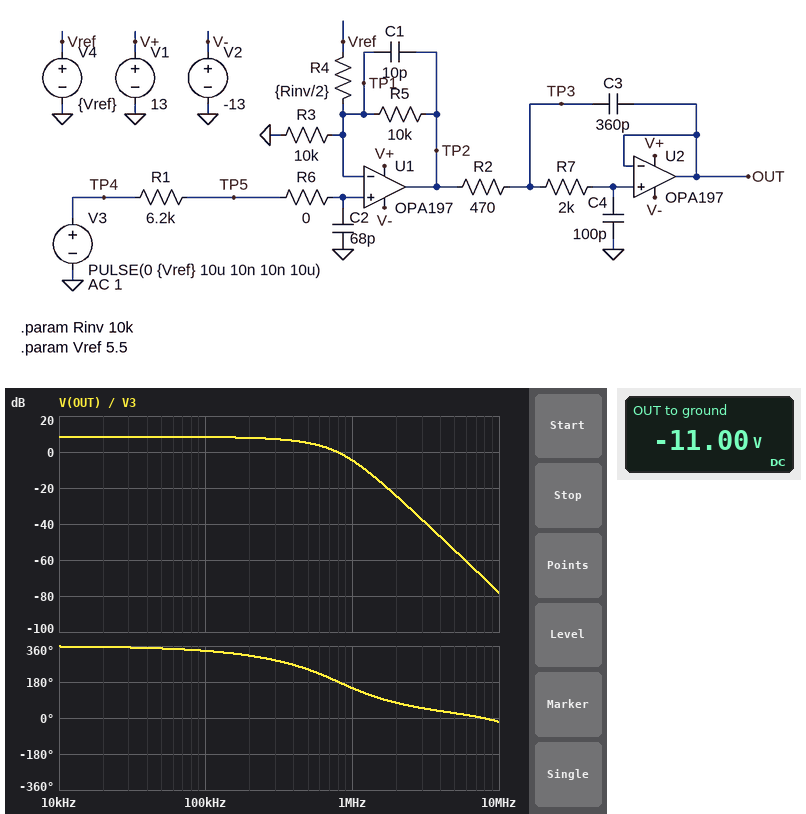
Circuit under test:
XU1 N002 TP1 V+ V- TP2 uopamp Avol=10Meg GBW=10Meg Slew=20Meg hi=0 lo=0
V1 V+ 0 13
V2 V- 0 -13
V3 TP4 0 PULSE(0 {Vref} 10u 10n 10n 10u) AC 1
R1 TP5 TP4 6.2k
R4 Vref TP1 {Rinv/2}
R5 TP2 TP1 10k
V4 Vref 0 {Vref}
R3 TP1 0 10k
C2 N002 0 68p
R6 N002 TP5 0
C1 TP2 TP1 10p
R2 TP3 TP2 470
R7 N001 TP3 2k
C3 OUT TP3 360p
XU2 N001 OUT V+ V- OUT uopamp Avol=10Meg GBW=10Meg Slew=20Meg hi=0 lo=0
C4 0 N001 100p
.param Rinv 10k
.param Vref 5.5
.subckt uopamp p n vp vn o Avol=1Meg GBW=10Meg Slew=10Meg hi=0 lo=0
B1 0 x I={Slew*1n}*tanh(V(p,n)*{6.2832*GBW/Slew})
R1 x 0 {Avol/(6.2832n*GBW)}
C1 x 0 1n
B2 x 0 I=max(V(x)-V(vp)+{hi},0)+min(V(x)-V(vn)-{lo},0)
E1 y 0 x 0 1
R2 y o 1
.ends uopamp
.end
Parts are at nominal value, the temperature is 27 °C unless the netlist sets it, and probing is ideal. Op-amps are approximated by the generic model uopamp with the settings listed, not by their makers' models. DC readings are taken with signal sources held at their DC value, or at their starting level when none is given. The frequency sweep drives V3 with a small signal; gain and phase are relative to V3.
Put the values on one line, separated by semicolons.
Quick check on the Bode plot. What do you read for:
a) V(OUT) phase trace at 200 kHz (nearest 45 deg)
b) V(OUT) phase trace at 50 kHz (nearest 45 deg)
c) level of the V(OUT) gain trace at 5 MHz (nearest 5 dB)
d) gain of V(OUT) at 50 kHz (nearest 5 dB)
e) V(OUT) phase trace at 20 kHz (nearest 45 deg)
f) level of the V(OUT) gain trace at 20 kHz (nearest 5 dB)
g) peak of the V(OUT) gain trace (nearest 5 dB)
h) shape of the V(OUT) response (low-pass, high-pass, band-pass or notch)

315 deg; 360 deg; -55 dB; 10 dB; 360 deg; 10 dB; 10 dB; low-pass
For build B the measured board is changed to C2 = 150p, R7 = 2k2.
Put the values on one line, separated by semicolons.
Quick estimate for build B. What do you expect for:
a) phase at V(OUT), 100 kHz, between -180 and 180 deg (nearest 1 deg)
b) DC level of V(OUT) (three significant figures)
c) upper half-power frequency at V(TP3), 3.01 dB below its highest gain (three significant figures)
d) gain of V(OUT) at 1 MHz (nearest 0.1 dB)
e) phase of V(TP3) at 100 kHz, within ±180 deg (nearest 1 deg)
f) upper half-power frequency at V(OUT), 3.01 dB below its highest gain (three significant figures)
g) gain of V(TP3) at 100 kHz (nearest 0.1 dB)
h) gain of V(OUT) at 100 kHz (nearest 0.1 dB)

-36 deg; -11.0 V; 280 kHz; -11.4 dB; -28 deg; 248 kHz; 7.9 dB; 7.8 dB
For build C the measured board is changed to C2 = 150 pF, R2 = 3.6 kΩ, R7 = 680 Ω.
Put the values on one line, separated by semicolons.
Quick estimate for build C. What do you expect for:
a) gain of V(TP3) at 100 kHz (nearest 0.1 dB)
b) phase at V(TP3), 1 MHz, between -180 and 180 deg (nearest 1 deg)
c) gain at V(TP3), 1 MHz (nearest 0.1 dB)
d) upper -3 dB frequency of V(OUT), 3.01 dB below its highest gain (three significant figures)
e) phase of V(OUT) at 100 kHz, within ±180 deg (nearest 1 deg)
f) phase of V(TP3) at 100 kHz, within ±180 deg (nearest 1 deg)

7.9 dB; 129 deg; -18.3 dB; 248 kHz; -42 deg; -39 deg
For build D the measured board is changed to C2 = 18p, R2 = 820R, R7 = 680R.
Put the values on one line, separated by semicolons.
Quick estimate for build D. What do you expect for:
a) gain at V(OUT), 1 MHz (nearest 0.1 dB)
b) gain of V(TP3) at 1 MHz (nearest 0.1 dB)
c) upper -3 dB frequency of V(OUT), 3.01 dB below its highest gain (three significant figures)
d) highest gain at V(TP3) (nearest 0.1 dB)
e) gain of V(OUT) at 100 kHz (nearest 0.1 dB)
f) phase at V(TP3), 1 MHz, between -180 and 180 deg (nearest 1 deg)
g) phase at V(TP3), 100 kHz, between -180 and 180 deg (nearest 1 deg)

5.1 dB; 5.9 dB; 979 kHz; 8.5 dB; 8.4 dB; -129 deg; -11 deg
